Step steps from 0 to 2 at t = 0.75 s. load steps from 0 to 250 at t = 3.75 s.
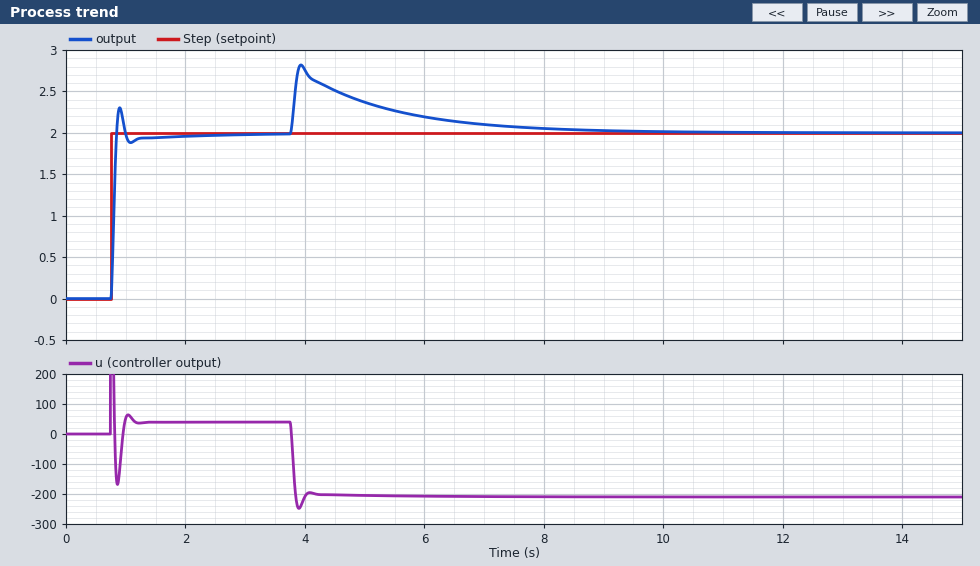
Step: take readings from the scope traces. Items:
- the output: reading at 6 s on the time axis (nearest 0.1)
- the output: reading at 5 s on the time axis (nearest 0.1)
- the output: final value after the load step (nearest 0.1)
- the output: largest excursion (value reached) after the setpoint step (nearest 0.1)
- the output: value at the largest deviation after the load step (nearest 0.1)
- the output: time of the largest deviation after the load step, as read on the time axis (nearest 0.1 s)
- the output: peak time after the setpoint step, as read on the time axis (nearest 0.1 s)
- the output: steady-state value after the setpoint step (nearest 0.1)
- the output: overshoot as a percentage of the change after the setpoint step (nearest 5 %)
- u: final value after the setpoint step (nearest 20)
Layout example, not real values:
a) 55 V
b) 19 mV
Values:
a) 2.2
b) 2.4
c) 2.0
d) 2.3
e) 2.8
f) 3.9 s
g) 0.9 s
h) 2.0
i) 15 %
j) 40
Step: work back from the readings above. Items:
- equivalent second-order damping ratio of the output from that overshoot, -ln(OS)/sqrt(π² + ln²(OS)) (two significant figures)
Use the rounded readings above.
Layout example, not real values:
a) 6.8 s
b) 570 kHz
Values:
a) 0.52
